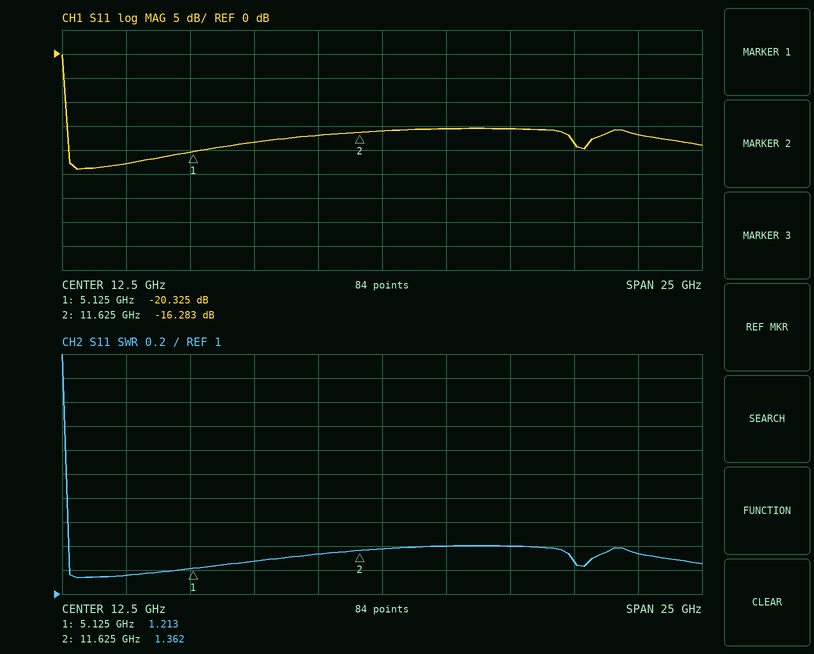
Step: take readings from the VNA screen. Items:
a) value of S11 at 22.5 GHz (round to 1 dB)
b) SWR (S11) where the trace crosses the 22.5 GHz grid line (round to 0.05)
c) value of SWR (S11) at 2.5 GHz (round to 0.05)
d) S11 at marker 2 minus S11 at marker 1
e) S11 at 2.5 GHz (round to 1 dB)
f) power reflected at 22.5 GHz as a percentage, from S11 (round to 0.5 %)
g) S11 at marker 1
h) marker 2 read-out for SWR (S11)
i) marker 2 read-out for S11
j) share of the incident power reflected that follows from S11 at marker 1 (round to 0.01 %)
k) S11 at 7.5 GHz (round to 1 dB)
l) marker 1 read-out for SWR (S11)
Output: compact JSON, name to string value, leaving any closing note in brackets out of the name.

{"value of S11 at 22.5 GHz": "-17 dB", "SWR (S11) where the trace crosses the 22.5 GHz grid line": "1.35", "value of SWR (S11) at 2.5 GHz": "1.15", "S11 at marker 2 minus S11 at marker 1": "4.042 dB", "S11 at 2.5 GHz": "-23 dB", "power reflected at 22.5 GHz as a percentage, from S11": "2.0 %", "S11 at marker 1": "-20.325 dB", "marker 2 read-out for SWR": "1.362", "marker 2 read-out for S11": "-16.283 dB", "share of the incident power reflected that follows from S11 at marker 1": "0.93 %", "S11 at 7.5 GHz": "-18 dB", "marker 1 read-out for SWR": "1.213"}
